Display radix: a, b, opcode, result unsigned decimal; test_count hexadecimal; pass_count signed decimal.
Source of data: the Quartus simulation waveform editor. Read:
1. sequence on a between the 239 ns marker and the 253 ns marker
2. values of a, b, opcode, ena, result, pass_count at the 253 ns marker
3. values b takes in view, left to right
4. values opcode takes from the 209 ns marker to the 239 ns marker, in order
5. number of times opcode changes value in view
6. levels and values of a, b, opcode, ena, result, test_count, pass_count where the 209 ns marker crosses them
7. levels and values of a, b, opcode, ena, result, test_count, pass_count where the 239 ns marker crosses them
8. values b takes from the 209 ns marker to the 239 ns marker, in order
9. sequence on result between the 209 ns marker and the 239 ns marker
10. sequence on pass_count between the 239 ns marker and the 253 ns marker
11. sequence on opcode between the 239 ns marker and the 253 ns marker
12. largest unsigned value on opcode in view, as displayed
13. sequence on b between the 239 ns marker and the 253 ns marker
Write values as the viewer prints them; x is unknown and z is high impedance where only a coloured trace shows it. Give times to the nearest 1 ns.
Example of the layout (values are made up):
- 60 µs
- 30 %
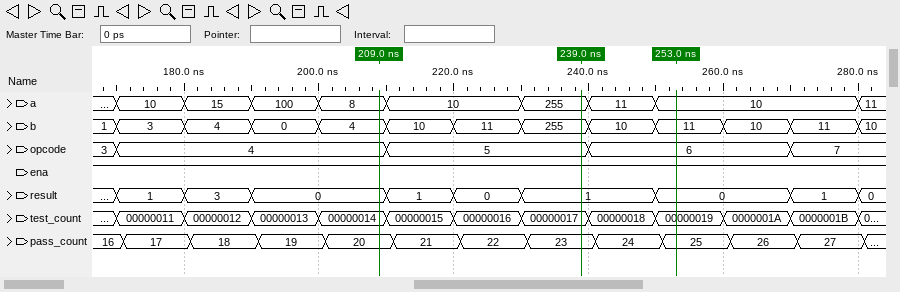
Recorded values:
- 255, 11, 10
- a=10, b=11, opcode=6, ena=1, result=0, pass_count=25
- 1, 3, 4, 0, 4, 10, 11, 255, 10, 11, 10, 11, 10
- 4, 5
- 4
- a=8, b=4, opcode=4, ena=1, result=0, test_count=00000014, pass_count=20
- a=255, b=255, opcode=5, ena=1, result=1, test_count=00000017, pass_count=23
- 4, 10, 11, 255
- 0, 1, 0, 1
- 23, 24, 25
- 5, 6
- 7
- 255, 10, 11
